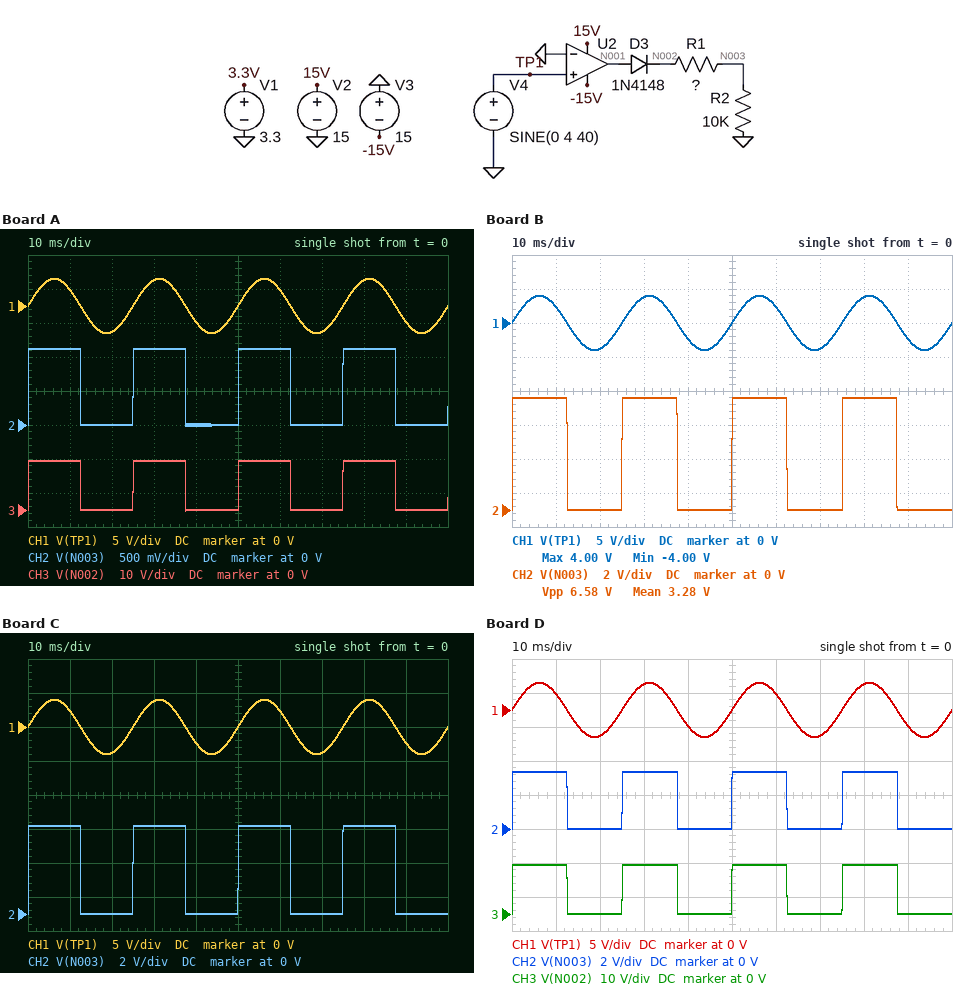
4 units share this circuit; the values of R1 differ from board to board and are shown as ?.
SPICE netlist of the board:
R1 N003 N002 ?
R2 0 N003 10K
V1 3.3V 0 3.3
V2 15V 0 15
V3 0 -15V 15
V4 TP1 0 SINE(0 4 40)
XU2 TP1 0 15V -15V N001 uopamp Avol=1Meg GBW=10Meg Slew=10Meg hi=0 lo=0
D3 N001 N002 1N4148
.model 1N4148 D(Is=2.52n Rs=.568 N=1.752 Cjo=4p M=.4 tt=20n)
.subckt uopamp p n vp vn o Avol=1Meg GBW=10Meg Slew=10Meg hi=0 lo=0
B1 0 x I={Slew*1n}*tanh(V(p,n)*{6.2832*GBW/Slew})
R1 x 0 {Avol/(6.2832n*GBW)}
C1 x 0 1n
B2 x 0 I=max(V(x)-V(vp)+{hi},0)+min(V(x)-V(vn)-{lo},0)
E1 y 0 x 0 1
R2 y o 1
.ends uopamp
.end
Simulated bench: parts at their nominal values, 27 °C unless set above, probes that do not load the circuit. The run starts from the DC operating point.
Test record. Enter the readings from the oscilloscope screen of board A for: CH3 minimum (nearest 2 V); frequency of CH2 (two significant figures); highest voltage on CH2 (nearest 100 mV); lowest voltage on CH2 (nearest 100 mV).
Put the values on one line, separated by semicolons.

0 V; 40 Hz; 1.1 V; 0 V
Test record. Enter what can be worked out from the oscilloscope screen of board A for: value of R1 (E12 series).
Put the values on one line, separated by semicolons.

120 kΩ
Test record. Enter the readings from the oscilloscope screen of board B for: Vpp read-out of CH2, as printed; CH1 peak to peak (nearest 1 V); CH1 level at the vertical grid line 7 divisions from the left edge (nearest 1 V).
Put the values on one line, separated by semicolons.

6.58 V; 8 V; -4 V
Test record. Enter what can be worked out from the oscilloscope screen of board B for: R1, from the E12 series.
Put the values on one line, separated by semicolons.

12 kΩ
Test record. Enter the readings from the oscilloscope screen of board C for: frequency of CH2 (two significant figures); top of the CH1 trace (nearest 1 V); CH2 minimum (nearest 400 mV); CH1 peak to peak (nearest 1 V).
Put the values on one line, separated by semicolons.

40 Hz; 4 V; 0 V; 8 V
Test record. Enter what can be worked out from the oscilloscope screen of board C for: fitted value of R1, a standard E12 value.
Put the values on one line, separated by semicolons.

18 kΩ
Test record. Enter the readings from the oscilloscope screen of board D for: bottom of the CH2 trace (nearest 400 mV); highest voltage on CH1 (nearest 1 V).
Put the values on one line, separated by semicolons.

0 V; 4 V
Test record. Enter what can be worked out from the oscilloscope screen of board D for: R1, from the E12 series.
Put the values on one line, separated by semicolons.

33 kΩ
